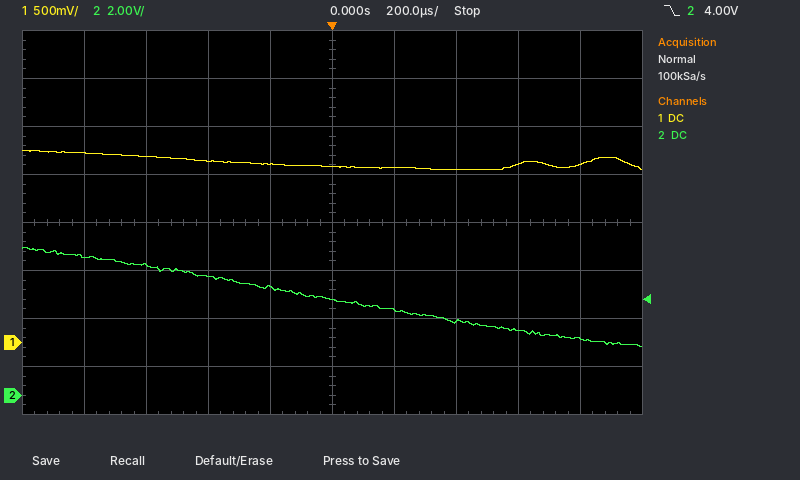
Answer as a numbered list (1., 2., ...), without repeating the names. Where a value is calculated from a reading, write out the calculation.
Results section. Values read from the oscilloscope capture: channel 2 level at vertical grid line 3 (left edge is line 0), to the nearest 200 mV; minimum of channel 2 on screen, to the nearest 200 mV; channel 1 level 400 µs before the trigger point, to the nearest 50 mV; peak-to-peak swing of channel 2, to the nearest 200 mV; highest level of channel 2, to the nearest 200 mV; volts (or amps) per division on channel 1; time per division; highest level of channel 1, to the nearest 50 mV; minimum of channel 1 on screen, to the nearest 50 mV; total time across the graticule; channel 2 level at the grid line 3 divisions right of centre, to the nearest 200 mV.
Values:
1. 5.0 V
2. 2.0 V
3. 1.90 V
4. 6.2 V − (2.0 V) = 4.2 V
5. 6.2 V
6. 500 mV
7. 200 µs
8. 2.00 V
9. 1.80 V
10. 2 ms
11. 2.8 V
